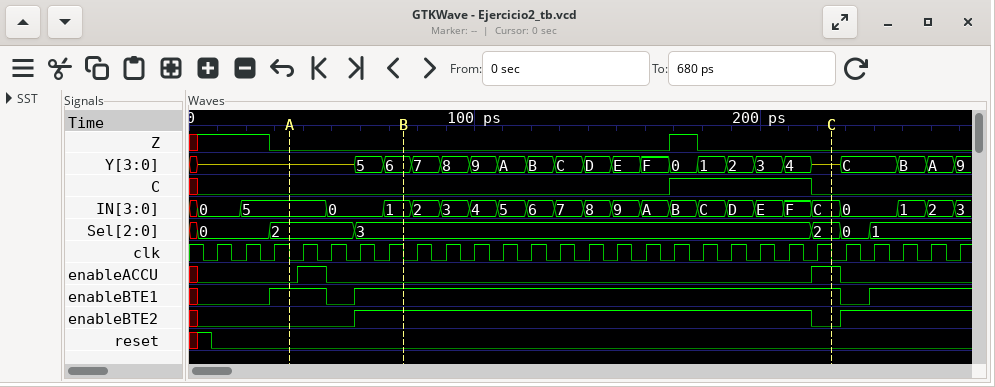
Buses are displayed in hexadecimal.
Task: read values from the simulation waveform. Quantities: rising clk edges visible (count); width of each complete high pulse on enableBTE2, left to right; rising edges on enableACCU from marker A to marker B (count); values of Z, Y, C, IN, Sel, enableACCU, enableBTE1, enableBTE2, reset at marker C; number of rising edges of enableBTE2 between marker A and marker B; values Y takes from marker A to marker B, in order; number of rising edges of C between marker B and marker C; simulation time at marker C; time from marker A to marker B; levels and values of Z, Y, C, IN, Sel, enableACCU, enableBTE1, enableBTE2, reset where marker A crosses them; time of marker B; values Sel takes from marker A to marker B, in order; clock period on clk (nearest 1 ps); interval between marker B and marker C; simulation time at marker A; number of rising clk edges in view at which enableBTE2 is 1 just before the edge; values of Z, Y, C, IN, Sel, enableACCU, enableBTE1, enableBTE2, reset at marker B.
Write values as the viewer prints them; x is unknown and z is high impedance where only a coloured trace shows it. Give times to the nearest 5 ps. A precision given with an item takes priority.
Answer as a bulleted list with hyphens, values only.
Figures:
- 27
- 160 ps
- 1
- Z=0, Y=z, C=0, IN=C, Sel=2, enableACCU=1, enableBTE1=1, enableBTE2=0, reset=0
- 1
- z, 5, 6
- 1
- 225 ps
- 40 ps
- Z=0, Y=z, C=0, IN=5, Sel=2, enableACCU=0, enableBTE1=1, enableBTE2=0, reset=0
- 75 ps
- 2, 3
- 10 ps
- 150 ps
- 35 ps
- 21
- Z=0, Y=6, C=0, IN=1, Sel=3, enableACCU=0, enableBTE1=1, enableBTE2=1, reset=0
